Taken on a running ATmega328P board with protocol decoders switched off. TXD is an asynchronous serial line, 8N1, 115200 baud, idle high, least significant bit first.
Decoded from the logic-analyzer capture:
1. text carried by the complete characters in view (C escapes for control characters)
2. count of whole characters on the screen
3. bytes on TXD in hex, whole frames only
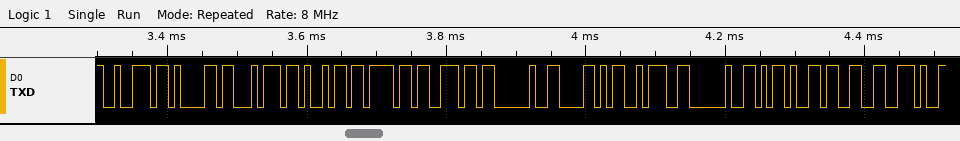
"ration X: -3."
13
72 61 74 69 6F 6E 20 58 3A 20 2D 33 2E
